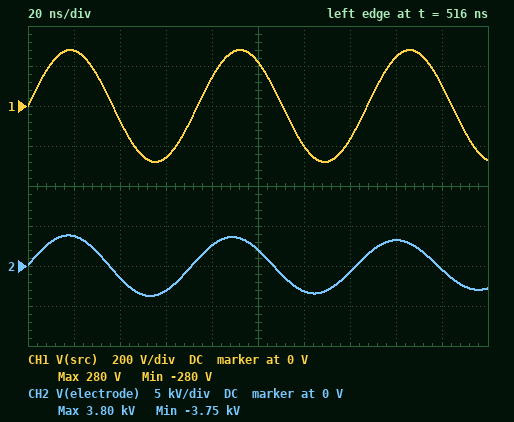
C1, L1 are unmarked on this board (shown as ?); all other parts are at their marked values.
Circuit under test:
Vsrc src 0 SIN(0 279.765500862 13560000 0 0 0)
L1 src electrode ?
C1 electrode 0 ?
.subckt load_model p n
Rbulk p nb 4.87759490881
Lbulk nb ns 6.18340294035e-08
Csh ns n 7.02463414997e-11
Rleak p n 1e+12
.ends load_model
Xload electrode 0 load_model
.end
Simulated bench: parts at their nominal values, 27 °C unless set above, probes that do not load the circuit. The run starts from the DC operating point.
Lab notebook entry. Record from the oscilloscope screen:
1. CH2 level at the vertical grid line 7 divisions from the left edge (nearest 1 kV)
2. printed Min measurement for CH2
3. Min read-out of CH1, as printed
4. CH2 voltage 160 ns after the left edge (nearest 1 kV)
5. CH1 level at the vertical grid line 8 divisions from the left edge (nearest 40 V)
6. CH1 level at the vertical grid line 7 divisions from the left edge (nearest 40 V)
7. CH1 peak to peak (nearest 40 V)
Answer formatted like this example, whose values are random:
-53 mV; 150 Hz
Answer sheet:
-1 kV; -3.75 kV; -280 V; 3 kV; 240 V; -160 V; 560 V
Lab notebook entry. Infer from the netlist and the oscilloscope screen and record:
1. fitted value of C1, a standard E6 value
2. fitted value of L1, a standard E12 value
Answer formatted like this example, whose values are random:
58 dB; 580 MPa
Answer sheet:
470 pF; 220 nH
